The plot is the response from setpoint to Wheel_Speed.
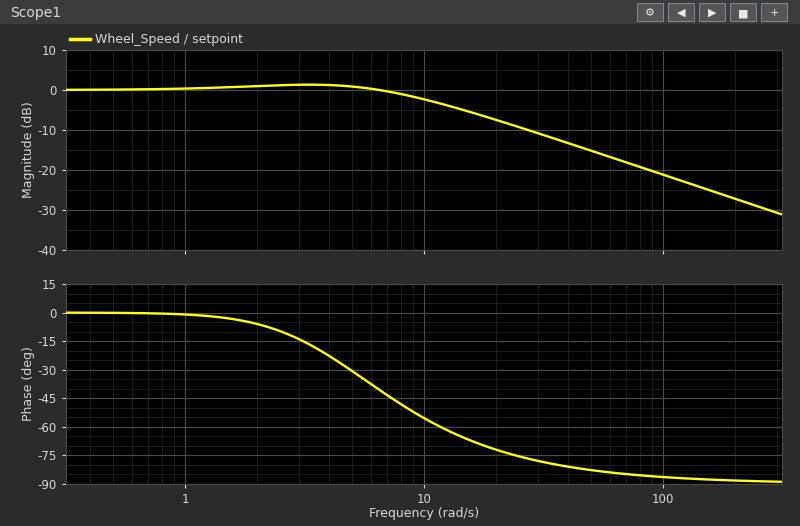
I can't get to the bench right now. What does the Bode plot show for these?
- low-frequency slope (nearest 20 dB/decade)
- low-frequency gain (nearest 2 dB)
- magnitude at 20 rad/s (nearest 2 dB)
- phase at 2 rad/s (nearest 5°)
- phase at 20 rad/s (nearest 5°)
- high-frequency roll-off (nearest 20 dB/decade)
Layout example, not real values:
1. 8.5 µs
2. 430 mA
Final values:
1. 0 dB/decade
2. 0 dB
3. -8 dB
4. -5°
5. -70°
6. -20 dB/decade
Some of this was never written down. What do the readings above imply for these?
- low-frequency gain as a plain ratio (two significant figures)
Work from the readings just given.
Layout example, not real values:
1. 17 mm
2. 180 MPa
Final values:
1. 1.0
